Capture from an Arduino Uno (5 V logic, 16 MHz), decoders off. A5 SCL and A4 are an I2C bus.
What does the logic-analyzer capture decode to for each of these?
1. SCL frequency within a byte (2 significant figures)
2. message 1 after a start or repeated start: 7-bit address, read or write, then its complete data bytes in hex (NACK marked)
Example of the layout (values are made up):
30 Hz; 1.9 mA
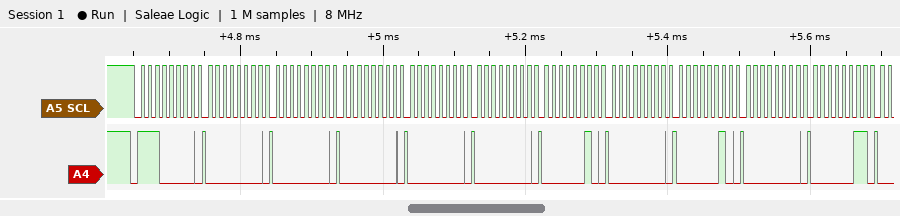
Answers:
100 kHz; 0x70 write: 00 00 00 00 00 02 00 02 00 03
